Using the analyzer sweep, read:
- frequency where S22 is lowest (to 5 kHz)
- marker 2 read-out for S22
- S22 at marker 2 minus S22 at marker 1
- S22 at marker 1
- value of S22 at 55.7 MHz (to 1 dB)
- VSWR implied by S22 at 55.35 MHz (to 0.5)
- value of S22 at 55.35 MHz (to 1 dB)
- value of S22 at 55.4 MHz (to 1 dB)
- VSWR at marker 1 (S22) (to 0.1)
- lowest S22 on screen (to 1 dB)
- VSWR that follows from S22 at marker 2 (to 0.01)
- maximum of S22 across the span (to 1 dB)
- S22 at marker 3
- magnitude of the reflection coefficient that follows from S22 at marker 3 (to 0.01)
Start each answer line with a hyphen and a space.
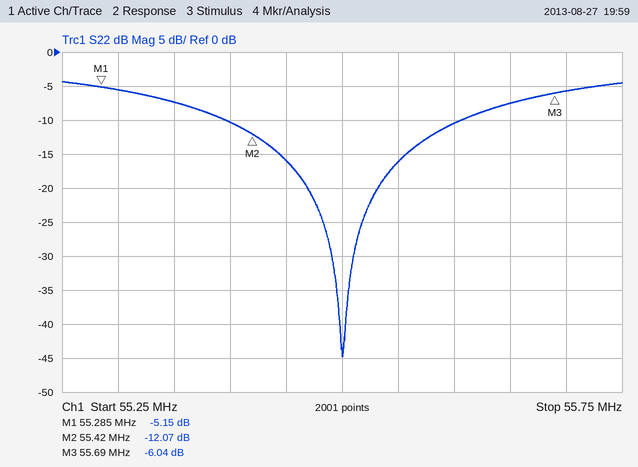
- 55.500 MHz
- -12.07 dB
- -6.92 dB
- -5.15 dB
- -6 dB
- 2.5
- -7 dB
- -10 dB
- 3.5
- -45 dB
- 1.66
- -4 dB
- -6.04 dB
- 0.50
